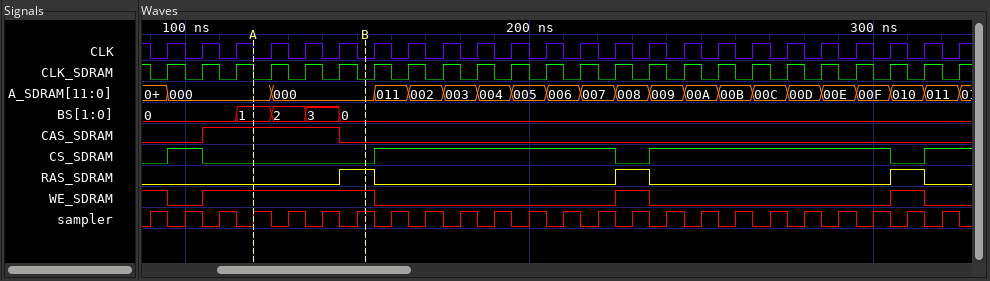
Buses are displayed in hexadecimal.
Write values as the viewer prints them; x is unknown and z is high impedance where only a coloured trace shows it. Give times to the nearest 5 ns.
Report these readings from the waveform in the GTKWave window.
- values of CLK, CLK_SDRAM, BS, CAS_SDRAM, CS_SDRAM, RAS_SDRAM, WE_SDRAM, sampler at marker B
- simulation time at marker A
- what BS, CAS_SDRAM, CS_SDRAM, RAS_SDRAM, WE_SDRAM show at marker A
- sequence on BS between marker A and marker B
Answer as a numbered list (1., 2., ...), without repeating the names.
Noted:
1. CLK=0, CLK_SDRAM=0, BS=0, CAS_SDRAM=0, CS_SDRAM=0, RAS_SDRAM=1, WE_SDRAM=1, sampler=1
2. 120 ns
3. BS=1, CAS_SDRAM=1, CS_SDRAM=0, RAS_SDRAM=0, WE_SDRAM=1
4. 1, 2, 3, 0
